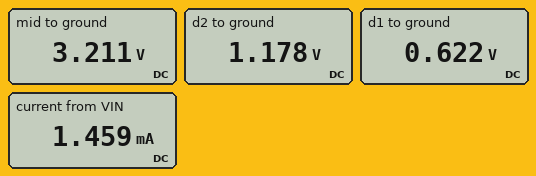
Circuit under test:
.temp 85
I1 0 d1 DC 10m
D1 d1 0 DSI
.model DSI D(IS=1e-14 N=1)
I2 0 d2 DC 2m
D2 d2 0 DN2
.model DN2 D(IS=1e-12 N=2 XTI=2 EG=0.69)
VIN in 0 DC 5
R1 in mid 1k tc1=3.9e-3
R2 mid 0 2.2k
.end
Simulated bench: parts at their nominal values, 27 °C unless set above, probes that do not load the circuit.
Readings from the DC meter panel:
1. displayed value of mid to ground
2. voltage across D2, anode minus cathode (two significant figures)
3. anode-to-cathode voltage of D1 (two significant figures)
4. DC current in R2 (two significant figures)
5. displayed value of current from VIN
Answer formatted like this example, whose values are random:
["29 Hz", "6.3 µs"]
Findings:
["3.211 V", "1.2 V", "620 mV", "1.5 mA", "1.459 mA"]
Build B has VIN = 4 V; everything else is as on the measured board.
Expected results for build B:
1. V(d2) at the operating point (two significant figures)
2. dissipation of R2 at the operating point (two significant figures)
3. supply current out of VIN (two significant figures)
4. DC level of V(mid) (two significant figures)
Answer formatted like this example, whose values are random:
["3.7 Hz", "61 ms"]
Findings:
["1.2 V", "3.0 mW", "1.2 mA", "2.6 V"]
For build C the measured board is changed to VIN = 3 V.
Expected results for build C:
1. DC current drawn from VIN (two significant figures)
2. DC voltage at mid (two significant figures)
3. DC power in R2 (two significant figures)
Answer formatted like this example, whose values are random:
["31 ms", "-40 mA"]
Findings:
["880 µA", "1.9 V", "1.7 mW"]
